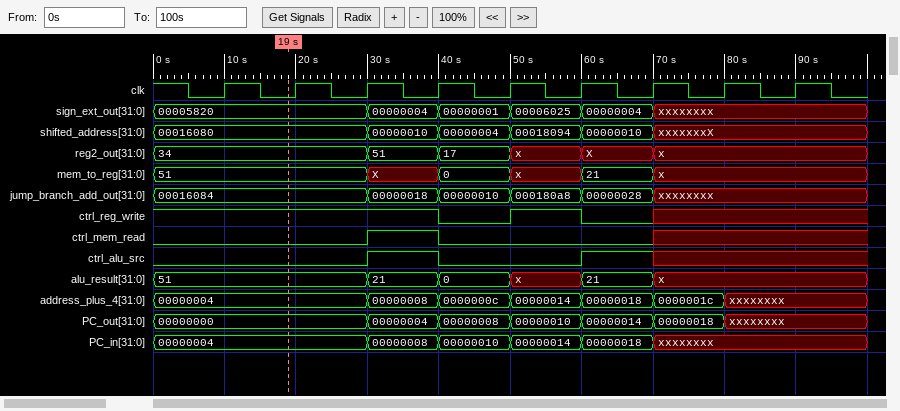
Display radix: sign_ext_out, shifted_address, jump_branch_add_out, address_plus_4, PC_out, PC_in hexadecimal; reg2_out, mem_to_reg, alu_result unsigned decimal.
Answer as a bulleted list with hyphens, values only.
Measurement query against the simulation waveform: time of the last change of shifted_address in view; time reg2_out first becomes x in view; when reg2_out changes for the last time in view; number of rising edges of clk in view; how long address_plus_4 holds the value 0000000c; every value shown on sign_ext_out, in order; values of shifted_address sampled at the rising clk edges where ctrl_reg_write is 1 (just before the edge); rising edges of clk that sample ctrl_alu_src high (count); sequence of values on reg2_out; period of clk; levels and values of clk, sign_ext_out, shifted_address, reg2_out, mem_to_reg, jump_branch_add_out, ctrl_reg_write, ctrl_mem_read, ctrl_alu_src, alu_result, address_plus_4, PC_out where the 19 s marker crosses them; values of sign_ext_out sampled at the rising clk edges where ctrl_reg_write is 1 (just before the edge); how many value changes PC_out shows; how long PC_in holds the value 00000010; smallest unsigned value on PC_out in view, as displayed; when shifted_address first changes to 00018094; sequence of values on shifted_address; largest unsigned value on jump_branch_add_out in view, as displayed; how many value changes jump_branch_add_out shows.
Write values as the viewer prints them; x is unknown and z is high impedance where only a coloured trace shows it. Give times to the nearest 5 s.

- 70 s
- 50 s
- 70 s
- 9
- 10 s
- 00005820, 00000004, 00000001, 00006025, 00000004, xxxxxxxx
- 00016080, 00016080, 00016080, 00000010, 00018094
- 2
- 34, 51, 17, x, X, x
- 10 s
- clk=0, sign_ext_out=00005820, shifted_address=00016080, reg2_out=34, mem_to_reg=51, jump_branch_add_out=00016084, ctrl_reg_write=1, ctrl_mem_read=0, ctrl_alu_src=0, alu_result=51, address_plus_4=00000004, PC_out=00000000
- 00005820, 00005820, 00005820, 00000004, 00006025
- 6
- 10 s
- 00000000
- 50 s
- 00016080, 00000010, 00000004, 00018094, 00000010, xxxxxxxX
- 000180a8
- 5
